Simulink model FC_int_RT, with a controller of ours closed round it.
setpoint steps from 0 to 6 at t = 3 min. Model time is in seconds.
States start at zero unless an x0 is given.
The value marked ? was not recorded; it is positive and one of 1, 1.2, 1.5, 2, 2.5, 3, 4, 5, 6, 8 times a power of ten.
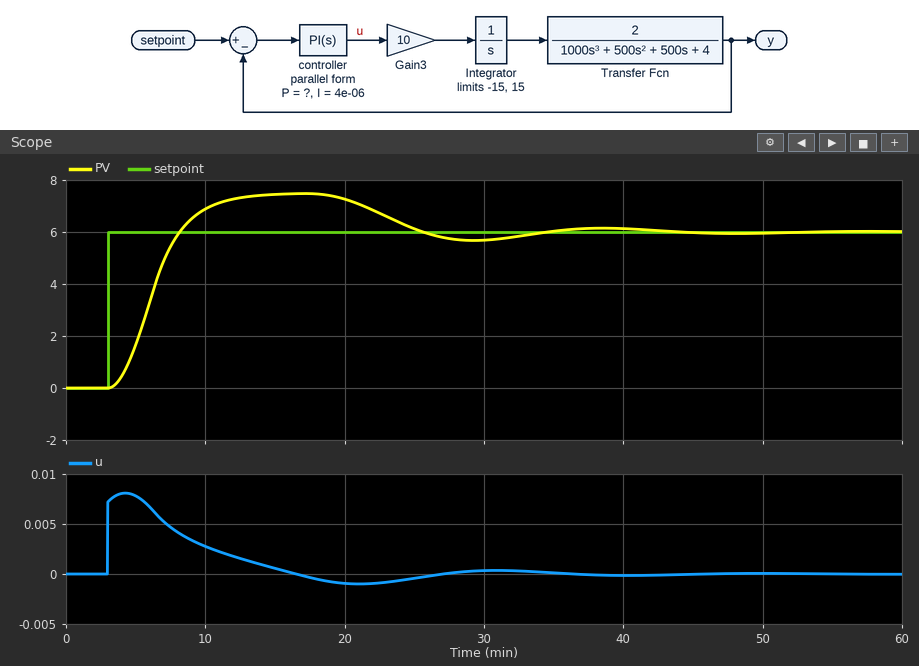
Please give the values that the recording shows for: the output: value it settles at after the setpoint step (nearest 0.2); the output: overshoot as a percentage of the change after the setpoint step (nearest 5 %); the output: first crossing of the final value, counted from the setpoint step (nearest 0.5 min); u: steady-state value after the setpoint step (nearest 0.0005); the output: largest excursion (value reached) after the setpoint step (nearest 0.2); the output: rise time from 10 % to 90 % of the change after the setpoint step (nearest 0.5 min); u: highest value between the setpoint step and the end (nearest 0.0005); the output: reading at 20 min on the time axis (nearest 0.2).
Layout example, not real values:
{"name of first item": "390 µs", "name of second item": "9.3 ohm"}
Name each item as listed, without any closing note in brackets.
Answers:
{"the output: value it settles at after the setpoint step": "6.0", "the output: overshoot as a percentage of the change after the setpoint step": "25 %", "the output: first crossing of the final value, counted from the setpoint step": "5.0 min", "u: steady-state value after the setpoint step": "0.0000", "the output: largest excursion (value reached) after the setpoint step": "7.4", "the output: rise time from 10 % to 90 % of the change after the setpoint step": "3.5 min", "u: highest value between the setpoint step and the end": "0.0080", "the output: reading at 20 min on the time axis": "7.2"}
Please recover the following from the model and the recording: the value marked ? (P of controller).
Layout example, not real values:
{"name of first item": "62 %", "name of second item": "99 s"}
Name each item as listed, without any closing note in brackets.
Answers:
{"the value marked ?": "0.0012"}
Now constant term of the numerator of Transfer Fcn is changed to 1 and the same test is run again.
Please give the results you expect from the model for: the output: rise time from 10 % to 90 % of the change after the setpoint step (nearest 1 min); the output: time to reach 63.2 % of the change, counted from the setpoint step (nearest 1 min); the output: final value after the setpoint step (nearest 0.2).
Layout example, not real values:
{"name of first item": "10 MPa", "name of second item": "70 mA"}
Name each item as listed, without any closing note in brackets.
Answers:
{"the output: rise time from 10 % to 90 % of the change after the setpoint step": "5 min", "the output: time to reach 63.2 % of the change, counted from the setpoint step": "4 min", "the output: final value after the setpoint step": "3.8"}
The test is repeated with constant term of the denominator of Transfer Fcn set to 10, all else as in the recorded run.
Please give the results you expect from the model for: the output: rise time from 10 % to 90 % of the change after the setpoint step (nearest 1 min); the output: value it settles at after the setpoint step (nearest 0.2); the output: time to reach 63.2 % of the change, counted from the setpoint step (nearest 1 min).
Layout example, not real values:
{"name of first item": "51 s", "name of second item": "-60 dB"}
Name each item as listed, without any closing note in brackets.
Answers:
{"the output: rise time from 10 % to 90 % of the change after the setpoint step": "3 min", "the output: value it settles at after the setpoint step": "3.0", "the output: time to reach 63.2 % of the change, counted from the setpoint step": "3 min"}
